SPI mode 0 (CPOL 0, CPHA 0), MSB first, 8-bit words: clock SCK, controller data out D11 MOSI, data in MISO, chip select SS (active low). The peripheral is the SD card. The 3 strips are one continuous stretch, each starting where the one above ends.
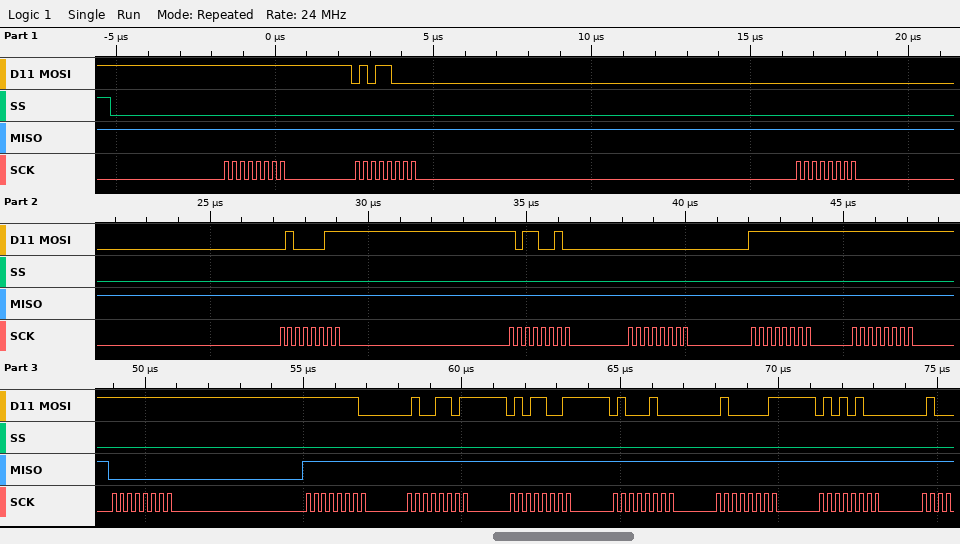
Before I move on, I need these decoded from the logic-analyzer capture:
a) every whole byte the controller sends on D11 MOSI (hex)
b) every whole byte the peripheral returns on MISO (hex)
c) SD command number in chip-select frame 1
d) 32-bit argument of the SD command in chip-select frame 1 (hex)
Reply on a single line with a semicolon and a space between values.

FF 58 00 43 B2 00 FF FF FF FE 4D 59 44 41 54; FF FF FF FF FF FF FF FF 00 FF FF FF FF FF FF; CMD24; 0x0043B200
